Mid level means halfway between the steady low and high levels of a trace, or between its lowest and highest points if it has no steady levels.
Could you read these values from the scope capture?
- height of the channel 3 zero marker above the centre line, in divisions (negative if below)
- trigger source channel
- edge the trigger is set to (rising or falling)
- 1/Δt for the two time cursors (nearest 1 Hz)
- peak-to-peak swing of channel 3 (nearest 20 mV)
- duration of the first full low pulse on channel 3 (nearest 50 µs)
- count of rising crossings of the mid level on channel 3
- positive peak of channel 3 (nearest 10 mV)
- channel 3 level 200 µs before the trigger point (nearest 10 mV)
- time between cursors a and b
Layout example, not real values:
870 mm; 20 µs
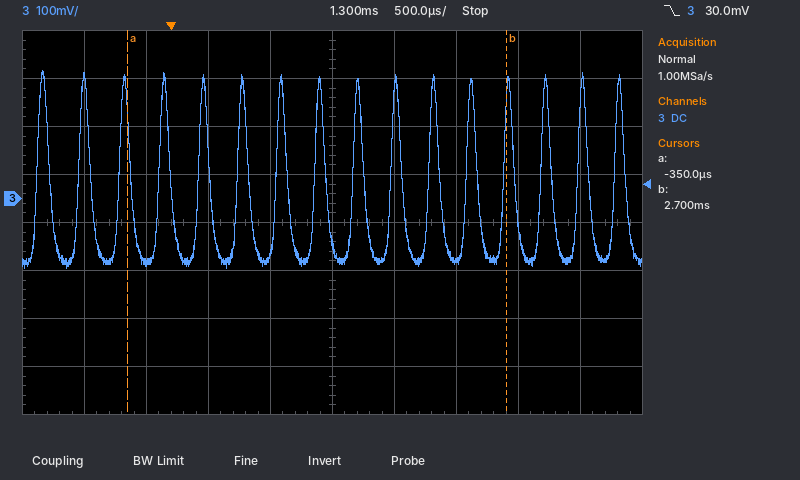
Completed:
+0.5 div; channel 3; falling; 328 Hz; 420 mV; 250 µs; 16; 270 mV; -130 mV; 3.05 ms
